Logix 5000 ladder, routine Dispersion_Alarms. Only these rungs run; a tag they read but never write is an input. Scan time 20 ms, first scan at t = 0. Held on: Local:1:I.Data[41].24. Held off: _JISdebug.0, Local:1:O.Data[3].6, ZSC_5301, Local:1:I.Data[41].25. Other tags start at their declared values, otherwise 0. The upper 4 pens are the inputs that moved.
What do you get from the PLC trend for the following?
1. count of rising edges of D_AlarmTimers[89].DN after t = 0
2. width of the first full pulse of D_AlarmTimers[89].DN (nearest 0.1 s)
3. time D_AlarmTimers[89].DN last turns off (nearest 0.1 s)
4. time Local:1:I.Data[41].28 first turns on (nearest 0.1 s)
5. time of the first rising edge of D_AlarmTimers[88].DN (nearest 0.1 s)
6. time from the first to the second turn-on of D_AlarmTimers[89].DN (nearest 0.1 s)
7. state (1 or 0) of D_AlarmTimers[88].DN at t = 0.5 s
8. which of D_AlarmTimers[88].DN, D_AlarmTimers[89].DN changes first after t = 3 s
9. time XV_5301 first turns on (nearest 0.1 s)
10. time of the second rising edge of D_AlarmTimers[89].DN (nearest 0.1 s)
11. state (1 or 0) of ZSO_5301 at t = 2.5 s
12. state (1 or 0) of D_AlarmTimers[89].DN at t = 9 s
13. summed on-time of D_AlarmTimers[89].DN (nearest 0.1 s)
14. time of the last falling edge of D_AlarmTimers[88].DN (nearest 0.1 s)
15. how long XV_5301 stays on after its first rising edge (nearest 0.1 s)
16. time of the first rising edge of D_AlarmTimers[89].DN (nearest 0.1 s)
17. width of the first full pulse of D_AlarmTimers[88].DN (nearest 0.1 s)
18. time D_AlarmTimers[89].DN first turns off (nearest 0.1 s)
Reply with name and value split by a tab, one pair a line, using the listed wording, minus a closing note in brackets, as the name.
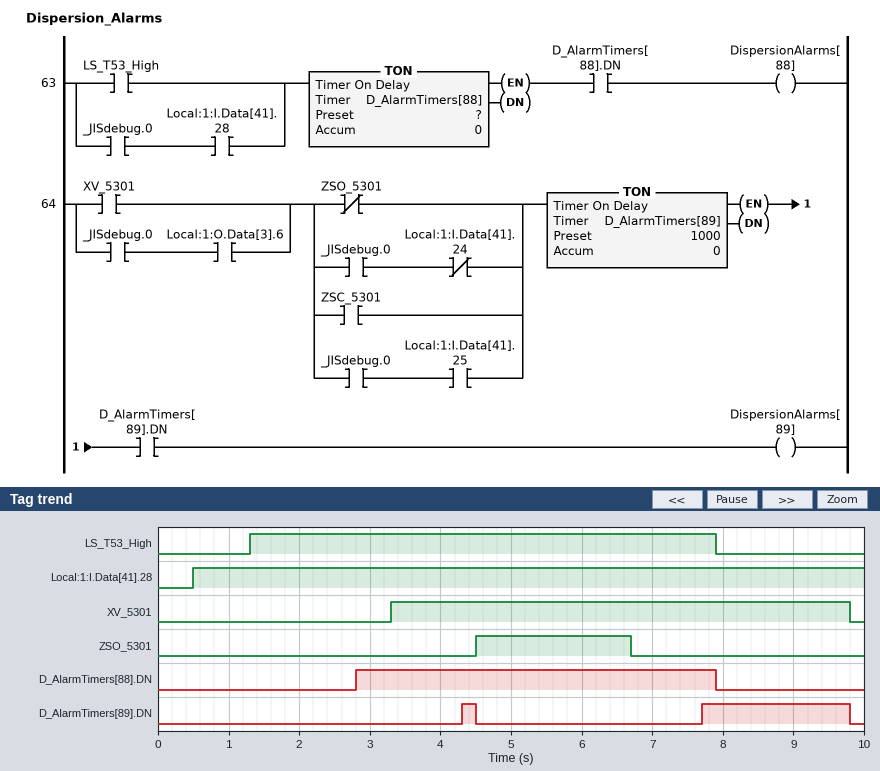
count of rising edges of D_AlarmTimers[89].DN after t = 0	2
width of the first full pulse of D_AlarmTimers[89].DN	0.2 s
time D_AlarmTimers[89].DN last turns off	9.8 s
time Local:1:I.Data[41].28 first turns on	0.5 s
time of the first rising edge of D_AlarmTimers[88].DN	2.8 s
time from the first to the second turn-on of D_AlarmTimers[89].DN	3.4 s
state (1 or 0) of D_AlarmTimers[88].DN at t = 0.5 s	0
which of D_AlarmTimers[88].DN, D_AlarmTimers[89].DN changes first after t = 3 s	D_AlarmTimers[89].DN
time XV_5301 first turns on	3.3 s
time of the second rising edge of D_AlarmTimers[89].DN	7.7 s
state (1 or 0) of ZSO_5301 at t = 2.5 s	0
state (1 or 0) of D_AlarmTimers[89].DN at t = 9 s	1
summed on-time of D_AlarmTimers[89].DN	2.3 s
time of the last falling edge of D_AlarmTimers[88].DN	7.9 s
how long XV_5301 stays on after its first rising edge	6.5 s
time of the first rising edge of D_AlarmTimers[89].DN	4.3 s
width of the first full pulse of D_AlarmTimers[88].DN	5.1 s
time D_AlarmTimers[89].DN first turns off	4.5 s
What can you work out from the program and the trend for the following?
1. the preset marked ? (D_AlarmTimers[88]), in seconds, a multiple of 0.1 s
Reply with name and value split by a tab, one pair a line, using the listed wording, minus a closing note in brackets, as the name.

the preset marked ? (D_AlarmTimers[88]), in seconds, a multiple of 0.1 s	1.5 s
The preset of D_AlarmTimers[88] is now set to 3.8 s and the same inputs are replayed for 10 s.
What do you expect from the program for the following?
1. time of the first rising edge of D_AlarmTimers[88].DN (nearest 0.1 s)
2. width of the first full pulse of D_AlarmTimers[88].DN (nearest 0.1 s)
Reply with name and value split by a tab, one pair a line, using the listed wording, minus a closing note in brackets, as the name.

time of the first rising edge of D_AlarmTimers[88].DN	5.1 s
width of the first full pulse of D_AlarmTimers[88].DN	2.8 s
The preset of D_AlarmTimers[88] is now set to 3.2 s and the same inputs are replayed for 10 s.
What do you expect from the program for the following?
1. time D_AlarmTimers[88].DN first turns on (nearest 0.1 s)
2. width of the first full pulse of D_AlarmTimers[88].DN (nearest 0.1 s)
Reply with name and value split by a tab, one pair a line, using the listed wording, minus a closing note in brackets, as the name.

time D_AlarmTimers[88].DN first turns on	4.5 s
width of the first full pulse of D_AlarmTimers[88].DN	3.4 s
